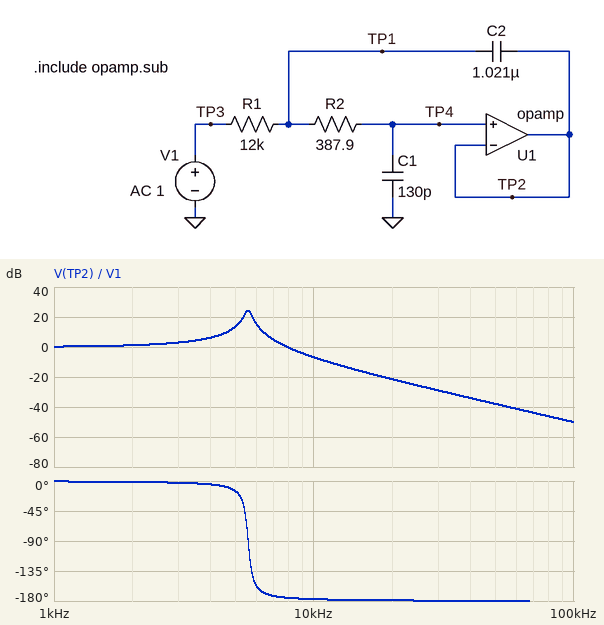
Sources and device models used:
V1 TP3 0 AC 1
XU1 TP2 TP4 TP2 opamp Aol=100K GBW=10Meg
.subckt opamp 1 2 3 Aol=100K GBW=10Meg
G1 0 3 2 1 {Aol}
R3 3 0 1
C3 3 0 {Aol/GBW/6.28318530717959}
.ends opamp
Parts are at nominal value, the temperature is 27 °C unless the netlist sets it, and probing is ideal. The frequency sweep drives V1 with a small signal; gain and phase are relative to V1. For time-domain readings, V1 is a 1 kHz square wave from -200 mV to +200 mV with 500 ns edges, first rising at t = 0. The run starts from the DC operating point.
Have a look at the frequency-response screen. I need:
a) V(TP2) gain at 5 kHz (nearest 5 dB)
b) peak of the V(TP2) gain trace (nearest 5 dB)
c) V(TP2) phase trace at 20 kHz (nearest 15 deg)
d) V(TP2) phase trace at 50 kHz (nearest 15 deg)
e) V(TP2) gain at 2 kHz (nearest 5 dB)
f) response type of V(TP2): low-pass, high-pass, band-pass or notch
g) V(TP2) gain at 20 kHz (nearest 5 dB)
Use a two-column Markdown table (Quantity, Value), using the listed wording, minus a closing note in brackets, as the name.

| Quantity | Value |
|---|---|
| V(TP2) gain at 5 kHz | 15 dB |
| peak of the V(TP2) gain trace | 25 dB |
| V(TP2) phase trace at 20 kHz | -180 deg |
| V(TP2) phase trace at 50 kHz | -180 deg |
| V(TP2) gain at 2 kHz | 0 dB |
| response type of V(TP2): low-pass, high-pass, band-pass or notch | low-pass |
| V(TP2) gain at 20 kHz | -20 dB |
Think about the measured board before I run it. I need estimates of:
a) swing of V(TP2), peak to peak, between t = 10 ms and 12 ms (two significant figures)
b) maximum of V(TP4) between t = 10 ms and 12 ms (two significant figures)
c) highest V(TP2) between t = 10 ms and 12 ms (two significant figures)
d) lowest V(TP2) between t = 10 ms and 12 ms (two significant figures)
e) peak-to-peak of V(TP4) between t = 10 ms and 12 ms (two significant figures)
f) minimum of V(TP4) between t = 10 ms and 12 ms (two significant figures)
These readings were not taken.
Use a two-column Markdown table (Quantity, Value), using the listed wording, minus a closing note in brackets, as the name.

| Quantity | Value |
|---|---|
| swing of V(TP2), peak to peak, between t = 10 ms and 12 ms | 980 mV |
| maximum of V(TP4) between t = 10 ms and 12 ms | 490 mV |
| highest V(TP2) between t = 10 ms and 12 ms | 490 mV |
| lowest V(TP2) between t = 10 ms and 12 ms | -490 mV |
| peak-to-peak of V(TP4) between t = 10 ms and 12 ms | 980 mV |
| minimum of V(TP4) between t = 10 ms and 12 ms | -490 mV |
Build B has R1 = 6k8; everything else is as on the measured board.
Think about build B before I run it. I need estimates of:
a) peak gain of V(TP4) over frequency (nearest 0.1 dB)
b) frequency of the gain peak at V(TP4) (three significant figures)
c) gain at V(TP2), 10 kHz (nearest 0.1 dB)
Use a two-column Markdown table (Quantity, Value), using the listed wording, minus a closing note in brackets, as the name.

| Quantity | Value |
|---|---|
| peak gain of V(TP4) over frequency | 26.6 dB |
| frequency of the gain peak at V(TP4) | 7.41 kHz |
| gain at V(TP2), 10 kHz | 1.7 dB |
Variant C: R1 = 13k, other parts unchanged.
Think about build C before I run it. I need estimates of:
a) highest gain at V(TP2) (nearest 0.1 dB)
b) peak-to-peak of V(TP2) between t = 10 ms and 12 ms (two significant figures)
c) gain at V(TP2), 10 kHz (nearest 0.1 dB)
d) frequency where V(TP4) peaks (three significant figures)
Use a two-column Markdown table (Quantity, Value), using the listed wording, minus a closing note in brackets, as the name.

| Quantity | Value |
|---|---|
| highest gain at V(TP2) | 24.0 dB |
| peak-to-peak of V(TP2) between t = 10 ms and 12 ms | 1.2 V |
| gain at V(TP2), 10 kHz | -7.9 dB |
| frequency where V(TP4) peaks | 5.36 kHz |
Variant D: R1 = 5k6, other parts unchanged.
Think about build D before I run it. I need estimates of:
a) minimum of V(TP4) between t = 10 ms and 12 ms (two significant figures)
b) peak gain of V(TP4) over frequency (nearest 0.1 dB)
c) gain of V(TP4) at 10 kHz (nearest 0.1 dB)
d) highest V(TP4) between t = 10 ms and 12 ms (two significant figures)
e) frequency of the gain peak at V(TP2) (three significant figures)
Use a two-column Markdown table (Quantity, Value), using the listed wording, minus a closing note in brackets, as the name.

| Quantity | Value |
|---|---|
| minimum of V(TP4) between t = 10 ms and 12 ms | -440 mV |
| peak gain of V(TP4) over frequency | 27.3 dB |
| gain of V(TP4) at 10 kHz | 6.0 dB |
| highest V(TP4) between t = 10 ms and 12 ms | 440 mV |
| frequency of the gain peak at V(TP2) | 8.17 kHz |
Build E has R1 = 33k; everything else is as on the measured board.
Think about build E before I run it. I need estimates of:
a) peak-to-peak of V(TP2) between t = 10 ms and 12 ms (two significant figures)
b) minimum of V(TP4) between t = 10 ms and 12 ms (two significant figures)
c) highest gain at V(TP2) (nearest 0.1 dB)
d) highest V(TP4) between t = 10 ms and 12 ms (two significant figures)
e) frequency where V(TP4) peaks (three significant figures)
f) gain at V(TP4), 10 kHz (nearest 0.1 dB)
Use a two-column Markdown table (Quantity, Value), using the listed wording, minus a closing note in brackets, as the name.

| Quantity | Value |
|---|---|
| peak-to-peak of V(TP2) between t = 10 ms and 12 ms | 1.2 V |
| minimum of V(TP4) between t = 10 ms and 12 ms | -580 mV |
| highest gain at V(TP2) | 20.1 dB |
| highest V(TP4) between t = 10 ms and 12 ms | 580 mV |
| frequency where V(TP4) peaks | 3.36 kHz |
| gain at V(TP4), 10 kHz | -17.9 dB |
